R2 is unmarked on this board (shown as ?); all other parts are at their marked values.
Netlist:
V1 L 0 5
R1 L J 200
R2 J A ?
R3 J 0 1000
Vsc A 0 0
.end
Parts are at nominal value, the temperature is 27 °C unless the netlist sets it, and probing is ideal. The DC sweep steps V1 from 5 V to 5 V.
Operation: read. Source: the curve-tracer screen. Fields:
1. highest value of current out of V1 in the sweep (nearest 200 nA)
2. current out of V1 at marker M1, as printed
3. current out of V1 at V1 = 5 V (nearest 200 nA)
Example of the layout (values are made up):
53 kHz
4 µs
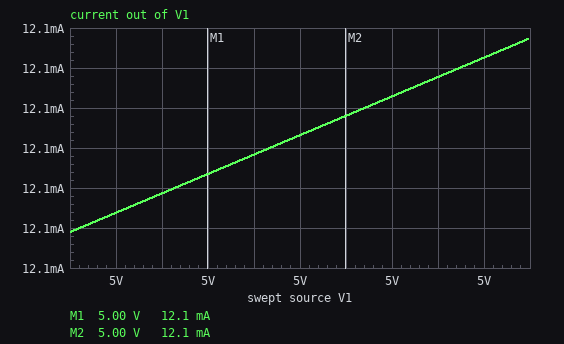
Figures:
12.1208 mA
12.1 mA
12.1188 mA
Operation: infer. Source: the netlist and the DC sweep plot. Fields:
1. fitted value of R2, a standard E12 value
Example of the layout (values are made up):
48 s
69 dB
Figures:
270 Ω
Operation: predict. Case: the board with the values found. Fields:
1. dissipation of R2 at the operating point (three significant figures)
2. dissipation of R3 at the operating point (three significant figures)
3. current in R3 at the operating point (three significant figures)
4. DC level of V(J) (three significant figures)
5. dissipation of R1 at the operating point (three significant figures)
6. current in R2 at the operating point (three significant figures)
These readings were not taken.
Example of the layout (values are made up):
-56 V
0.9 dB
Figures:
24.6 mW
6.64 mW
2.58 mA
2.58 V
29.4 mW
9.54 mA
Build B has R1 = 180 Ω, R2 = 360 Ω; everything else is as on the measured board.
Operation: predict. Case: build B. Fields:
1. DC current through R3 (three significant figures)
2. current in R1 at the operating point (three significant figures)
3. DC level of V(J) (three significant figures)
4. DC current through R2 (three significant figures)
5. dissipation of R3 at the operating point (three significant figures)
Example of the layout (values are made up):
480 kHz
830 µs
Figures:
2.98 mA
11.2 mA
2.98 V
8.27 mA
8.86 mW
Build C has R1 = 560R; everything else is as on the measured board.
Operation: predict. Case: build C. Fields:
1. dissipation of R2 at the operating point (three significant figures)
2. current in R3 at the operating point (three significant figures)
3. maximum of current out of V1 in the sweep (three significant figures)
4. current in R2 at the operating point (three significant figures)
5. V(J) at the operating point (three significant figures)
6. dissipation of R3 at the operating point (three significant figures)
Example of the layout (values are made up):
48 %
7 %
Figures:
7.01 mW
1.38 mA
6.47 mA
5.10 mA
1.38 V
1.89 mW
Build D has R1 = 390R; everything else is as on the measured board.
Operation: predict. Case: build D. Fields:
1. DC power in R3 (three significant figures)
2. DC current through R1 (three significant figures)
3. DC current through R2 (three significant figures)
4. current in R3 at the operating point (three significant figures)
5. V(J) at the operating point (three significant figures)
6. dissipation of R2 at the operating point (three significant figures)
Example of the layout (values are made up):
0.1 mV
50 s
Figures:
3.11 mW
8.30 mA
6.53 mA
1.76 mA
1.76 V
11.5 mW
